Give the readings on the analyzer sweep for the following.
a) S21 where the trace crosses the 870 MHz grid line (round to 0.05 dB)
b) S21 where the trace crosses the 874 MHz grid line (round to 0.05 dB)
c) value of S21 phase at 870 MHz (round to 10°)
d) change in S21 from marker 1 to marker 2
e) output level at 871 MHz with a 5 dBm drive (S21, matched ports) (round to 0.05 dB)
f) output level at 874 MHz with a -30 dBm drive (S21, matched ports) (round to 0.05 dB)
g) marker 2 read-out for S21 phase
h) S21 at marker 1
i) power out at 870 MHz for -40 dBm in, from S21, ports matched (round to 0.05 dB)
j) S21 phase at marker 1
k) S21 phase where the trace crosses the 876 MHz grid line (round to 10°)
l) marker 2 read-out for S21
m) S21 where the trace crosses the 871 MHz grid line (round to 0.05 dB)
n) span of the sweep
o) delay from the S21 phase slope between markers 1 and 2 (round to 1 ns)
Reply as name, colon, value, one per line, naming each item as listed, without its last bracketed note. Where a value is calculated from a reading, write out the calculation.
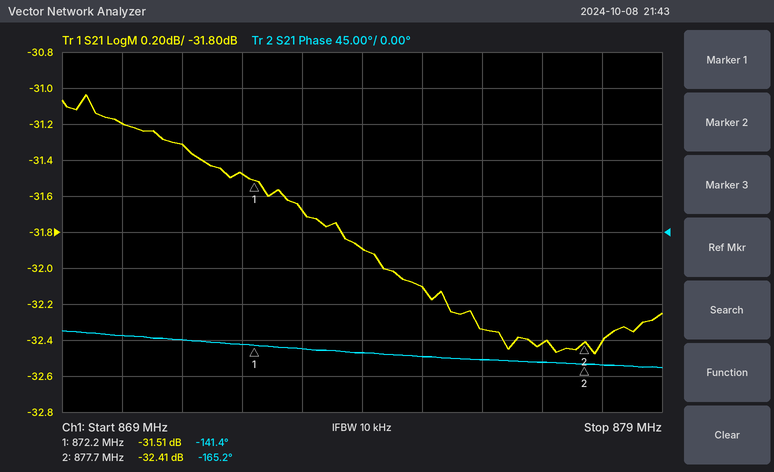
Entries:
S21 where the trace crosses the 870 MHz grid line: -31.20 dB
S21 where the trace crosses the 874 MHz grid line: -31.90 dB
value of S21 phase at 870 MHz: -130°
change in S21 from marker 1 to marker 2: -32.41 − (-31.51) = -0.90 dB
output level at 871 MHz with a 5 dBm drive (S21, matched ports): 5 dBm + (-31.30 dB) = -26.30 dBm
output level at 874 MHz with a -30 dBm drive (S21, matched ports): -30 dBm + (-31.90 dB) = -61.90 dBm
marker 2 read-out for S21 phase: -165.2°
S21 at marker 1: -31.51 dB
power out at 870 MHz for -40 dBm in, from S21, ports matched: -40 dBm + (-31.20 dB) = -71.20 dBm
S21 phase at marker 1: -141.4°
S21 phase where the trace crosses the 876 MHz grid line: -160°
marker 2 read-out for S21: -32.41 dB
S21 where the trace crosses the 871 MHz grid line: -31.30 dB
span of the sweep: 10 MHz
delay from the S21 phase slope between markers 1 and 2: −(-165.2° − (-141.4°))/(360° × 5.5 MHz) ≈ 12 ns
